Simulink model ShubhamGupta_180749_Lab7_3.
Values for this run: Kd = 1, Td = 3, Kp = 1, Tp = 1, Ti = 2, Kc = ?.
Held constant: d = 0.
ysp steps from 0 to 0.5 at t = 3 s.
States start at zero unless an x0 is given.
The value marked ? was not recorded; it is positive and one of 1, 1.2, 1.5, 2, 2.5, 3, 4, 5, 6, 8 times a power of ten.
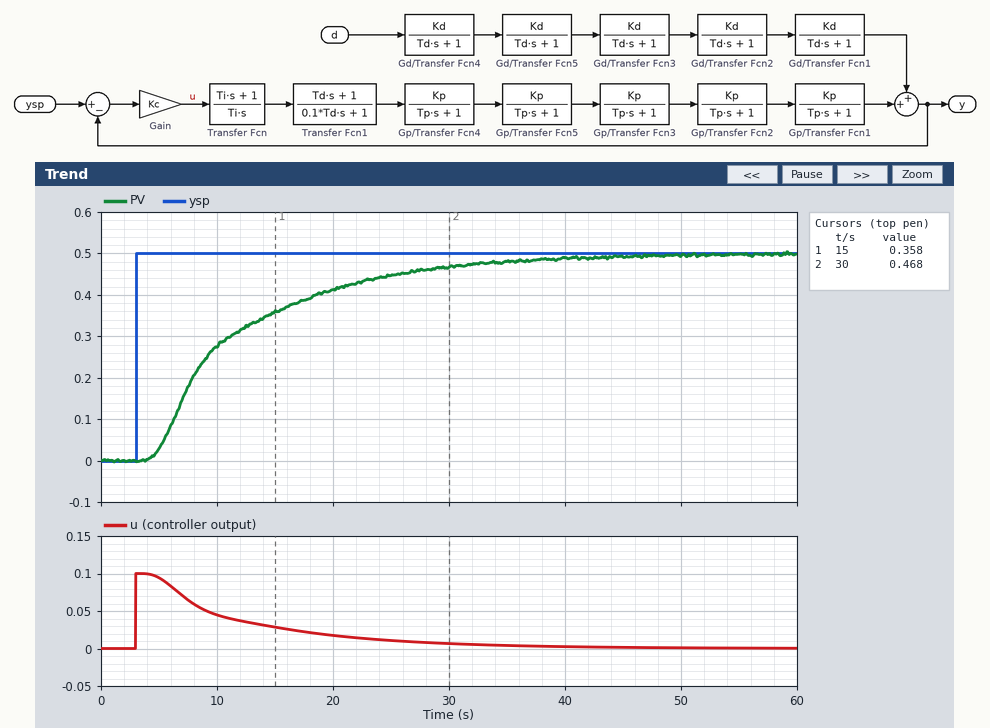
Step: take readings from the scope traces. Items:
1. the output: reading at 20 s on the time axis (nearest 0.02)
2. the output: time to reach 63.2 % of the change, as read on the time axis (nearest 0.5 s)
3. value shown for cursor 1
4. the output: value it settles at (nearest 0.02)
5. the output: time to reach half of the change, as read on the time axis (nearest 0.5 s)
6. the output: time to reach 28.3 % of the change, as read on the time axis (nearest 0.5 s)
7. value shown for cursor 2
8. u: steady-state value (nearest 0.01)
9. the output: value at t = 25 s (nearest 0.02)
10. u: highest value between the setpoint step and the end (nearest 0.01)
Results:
0.42
12.0 s
0.358
0.50
9.0 s
7.0 s
0.468
0.00
0.44
0.10
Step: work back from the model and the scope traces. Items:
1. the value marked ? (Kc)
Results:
0.2
